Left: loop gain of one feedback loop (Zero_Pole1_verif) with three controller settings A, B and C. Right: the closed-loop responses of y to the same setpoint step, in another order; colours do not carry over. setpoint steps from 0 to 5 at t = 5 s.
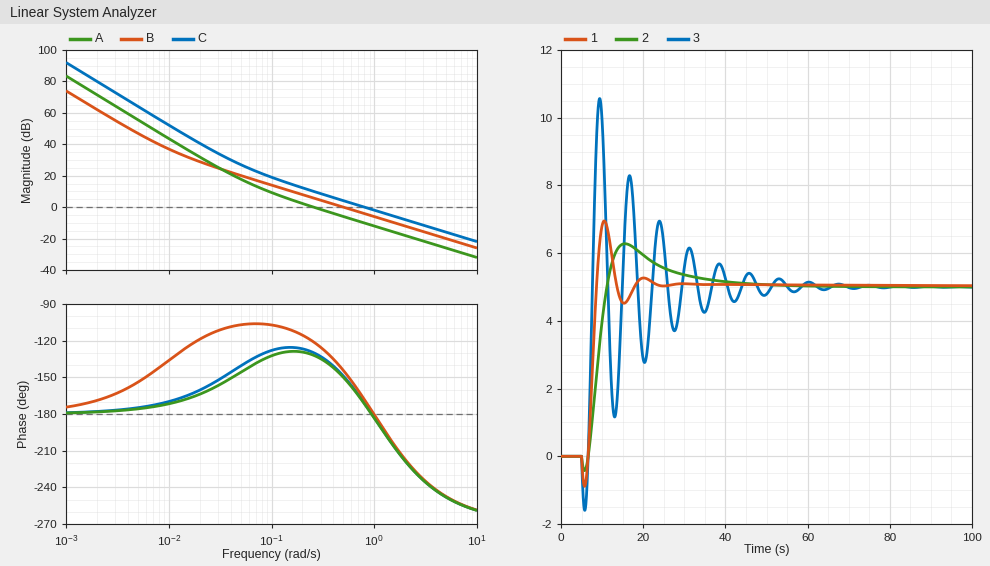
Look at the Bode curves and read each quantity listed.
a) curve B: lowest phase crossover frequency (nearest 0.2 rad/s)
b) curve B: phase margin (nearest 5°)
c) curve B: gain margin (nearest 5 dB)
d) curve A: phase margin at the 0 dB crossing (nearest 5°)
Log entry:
1.0 rad/s
35°
5 dB
50°
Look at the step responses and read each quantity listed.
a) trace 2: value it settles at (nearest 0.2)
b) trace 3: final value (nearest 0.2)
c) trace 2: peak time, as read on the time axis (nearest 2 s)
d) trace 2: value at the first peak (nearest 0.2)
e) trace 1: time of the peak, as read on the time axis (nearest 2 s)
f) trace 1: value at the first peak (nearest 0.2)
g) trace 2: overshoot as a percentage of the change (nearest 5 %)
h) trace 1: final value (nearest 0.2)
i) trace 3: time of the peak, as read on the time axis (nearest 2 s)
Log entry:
5.0
5.0
16 s
6.2
10 s
7.0
25 %
5.0
10 s
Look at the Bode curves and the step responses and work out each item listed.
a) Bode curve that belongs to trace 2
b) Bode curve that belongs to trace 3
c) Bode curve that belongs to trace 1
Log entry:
A
C
B
